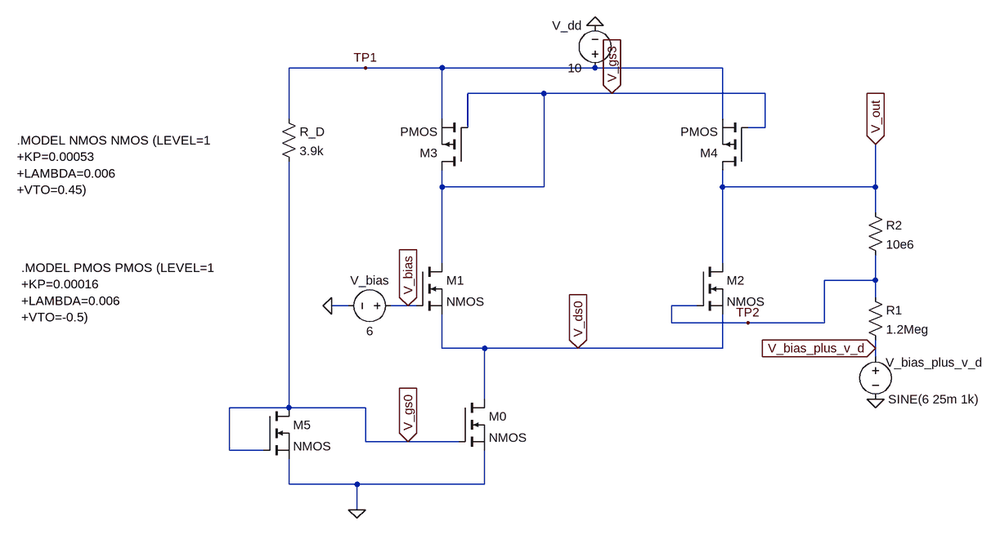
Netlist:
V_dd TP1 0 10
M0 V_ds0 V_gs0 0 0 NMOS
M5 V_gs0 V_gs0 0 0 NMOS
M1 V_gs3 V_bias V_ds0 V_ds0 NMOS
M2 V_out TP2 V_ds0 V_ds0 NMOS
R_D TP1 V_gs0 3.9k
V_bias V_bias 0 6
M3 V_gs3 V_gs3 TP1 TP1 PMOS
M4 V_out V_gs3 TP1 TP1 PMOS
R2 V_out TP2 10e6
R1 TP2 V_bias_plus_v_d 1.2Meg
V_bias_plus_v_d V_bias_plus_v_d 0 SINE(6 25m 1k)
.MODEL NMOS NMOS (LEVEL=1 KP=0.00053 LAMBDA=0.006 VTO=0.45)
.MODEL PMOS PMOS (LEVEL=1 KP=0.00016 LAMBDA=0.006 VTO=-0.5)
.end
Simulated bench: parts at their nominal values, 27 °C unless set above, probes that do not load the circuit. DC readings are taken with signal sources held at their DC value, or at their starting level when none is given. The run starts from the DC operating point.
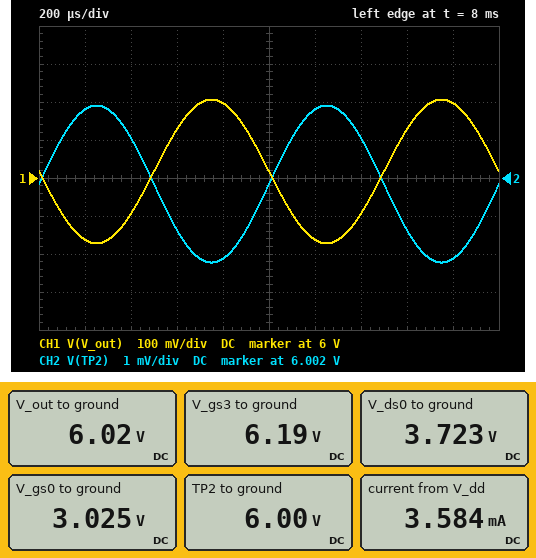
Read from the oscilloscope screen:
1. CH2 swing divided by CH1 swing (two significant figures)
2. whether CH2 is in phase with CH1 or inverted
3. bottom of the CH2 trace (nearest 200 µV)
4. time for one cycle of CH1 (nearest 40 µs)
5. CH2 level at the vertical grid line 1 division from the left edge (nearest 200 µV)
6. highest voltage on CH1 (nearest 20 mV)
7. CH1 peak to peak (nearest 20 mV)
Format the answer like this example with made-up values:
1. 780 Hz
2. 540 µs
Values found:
1. 0.011
2. inverted
3. 5.9998 V
4. 1.00 ms
5. 6.0038 V
6. 6.20 V
7. 380 mV
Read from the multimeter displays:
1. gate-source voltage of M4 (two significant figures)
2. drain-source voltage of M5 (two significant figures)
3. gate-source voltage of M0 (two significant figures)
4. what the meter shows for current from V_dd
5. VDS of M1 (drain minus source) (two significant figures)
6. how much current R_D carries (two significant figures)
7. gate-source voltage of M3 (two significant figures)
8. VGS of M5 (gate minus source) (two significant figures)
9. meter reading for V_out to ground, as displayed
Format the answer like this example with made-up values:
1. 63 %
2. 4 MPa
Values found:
1. -3.8 V
2. 3.0 V
3. 3.0 V
4. 3.584 mA
5. 2.5 V
6. 1.8 mA
7. -3.8 V
8. 3.0 V
9. 6.02 V
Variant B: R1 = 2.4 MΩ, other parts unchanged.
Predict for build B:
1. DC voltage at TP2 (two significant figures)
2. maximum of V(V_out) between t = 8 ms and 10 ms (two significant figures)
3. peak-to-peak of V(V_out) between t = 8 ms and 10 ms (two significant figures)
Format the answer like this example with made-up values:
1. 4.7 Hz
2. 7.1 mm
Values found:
1. 6.0 V
2. 6.1 V
3. 200 mV
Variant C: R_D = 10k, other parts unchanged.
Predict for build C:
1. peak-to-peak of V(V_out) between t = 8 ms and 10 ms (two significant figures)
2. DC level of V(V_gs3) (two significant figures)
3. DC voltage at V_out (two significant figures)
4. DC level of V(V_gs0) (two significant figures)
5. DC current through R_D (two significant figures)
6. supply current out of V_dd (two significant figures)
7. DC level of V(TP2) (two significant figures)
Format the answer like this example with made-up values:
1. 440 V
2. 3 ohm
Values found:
1. 390 mV
2. 7.3 V
3. 6.1 V
4. 2.2 V
5. 780 µA
6. 1.6 mA
7. 6.0 V
